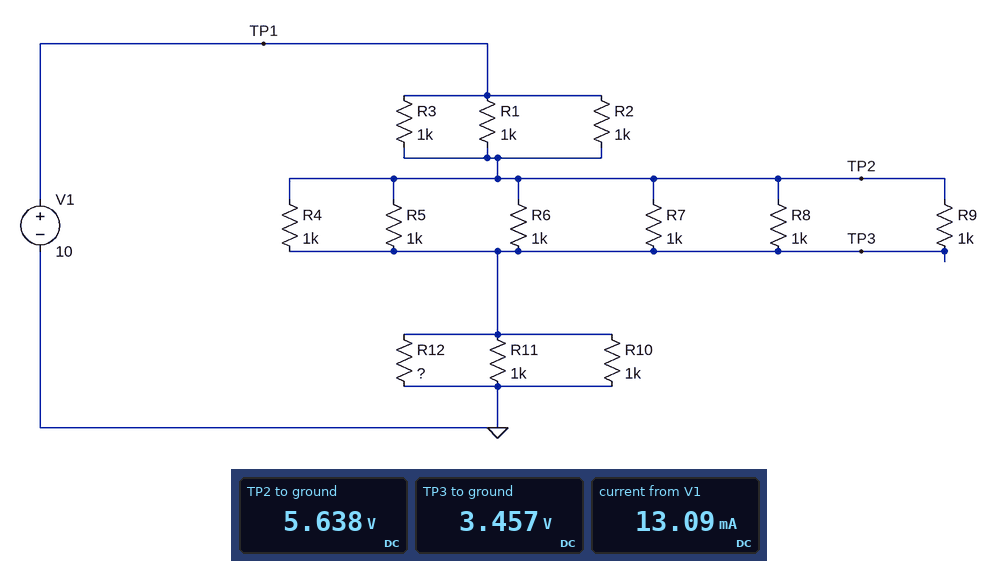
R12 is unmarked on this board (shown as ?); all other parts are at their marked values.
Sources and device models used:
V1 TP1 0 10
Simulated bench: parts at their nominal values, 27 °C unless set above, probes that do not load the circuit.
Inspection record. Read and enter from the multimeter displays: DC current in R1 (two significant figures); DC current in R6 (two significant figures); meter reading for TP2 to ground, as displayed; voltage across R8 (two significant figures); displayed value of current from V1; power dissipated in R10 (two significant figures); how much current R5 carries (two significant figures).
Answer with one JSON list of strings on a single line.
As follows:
["4.4 mA", "2.2 mA", "5.638 V", "2.2 V", "13.09 mA", "12 mW", "2.2 mA"]
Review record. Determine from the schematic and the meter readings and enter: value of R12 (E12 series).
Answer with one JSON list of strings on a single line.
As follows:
["560 Ω"]
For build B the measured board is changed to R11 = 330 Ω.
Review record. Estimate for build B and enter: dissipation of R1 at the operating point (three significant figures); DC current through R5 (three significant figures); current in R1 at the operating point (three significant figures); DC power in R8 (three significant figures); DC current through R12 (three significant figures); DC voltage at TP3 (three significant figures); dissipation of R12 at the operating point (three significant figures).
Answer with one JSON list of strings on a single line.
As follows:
["24.6 mW", "2.48 mA", "4.96 mA", "6.15 mW", "4.57 mA", "2.56 V", "11.7 mW"]
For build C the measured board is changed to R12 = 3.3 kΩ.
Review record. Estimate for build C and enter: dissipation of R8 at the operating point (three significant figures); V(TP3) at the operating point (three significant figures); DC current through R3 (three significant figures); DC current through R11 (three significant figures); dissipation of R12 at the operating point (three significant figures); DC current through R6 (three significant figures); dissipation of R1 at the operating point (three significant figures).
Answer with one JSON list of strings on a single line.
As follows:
["3.18 mW", "4.65 V", "3.57 mA", "4.65 mA", "6.55 mW", "1.78 mA", "12.7 mW"]
